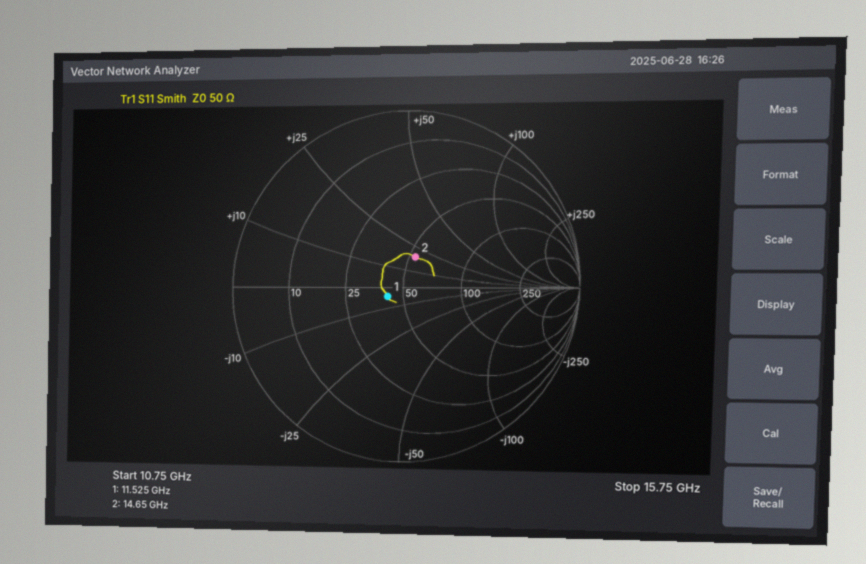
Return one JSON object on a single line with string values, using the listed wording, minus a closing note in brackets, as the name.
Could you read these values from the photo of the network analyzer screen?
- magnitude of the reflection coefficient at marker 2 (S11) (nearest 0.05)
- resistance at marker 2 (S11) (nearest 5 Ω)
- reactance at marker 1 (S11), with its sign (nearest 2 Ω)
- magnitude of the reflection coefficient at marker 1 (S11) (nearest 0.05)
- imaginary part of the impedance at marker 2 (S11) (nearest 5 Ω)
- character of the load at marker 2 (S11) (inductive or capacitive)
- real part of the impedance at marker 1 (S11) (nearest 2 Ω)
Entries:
{"magnitude of the reflection coefficient at marker 2 (S11)": "0.20", "resistance at marker 2 (S11)": "55 Ω", "reactance at marker 1 (S11), with its sign": "-4 Ω", "magnitude of the reflection coefficient at marker 1 (S11)": "0.10", "imaginary part of the impedance at marker 2 (S11)": "+20 Ω", "character of the load at marker 2 (S11)": "inductive", "real part of the impedance at marker 1 (S11)": "42 Ω"}
